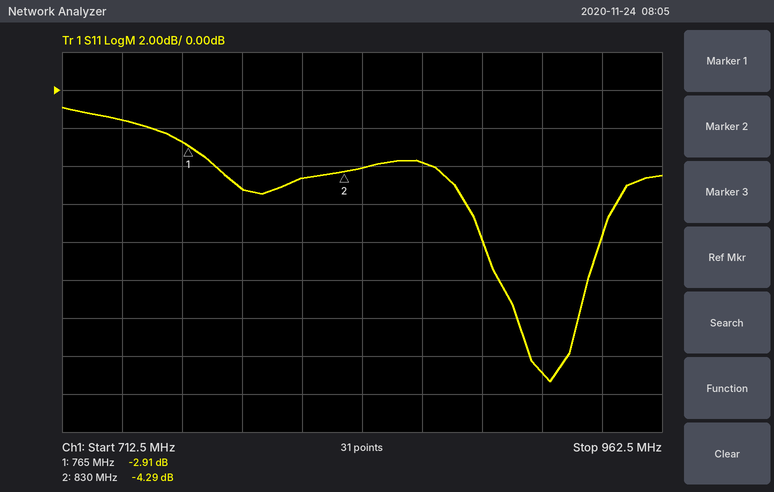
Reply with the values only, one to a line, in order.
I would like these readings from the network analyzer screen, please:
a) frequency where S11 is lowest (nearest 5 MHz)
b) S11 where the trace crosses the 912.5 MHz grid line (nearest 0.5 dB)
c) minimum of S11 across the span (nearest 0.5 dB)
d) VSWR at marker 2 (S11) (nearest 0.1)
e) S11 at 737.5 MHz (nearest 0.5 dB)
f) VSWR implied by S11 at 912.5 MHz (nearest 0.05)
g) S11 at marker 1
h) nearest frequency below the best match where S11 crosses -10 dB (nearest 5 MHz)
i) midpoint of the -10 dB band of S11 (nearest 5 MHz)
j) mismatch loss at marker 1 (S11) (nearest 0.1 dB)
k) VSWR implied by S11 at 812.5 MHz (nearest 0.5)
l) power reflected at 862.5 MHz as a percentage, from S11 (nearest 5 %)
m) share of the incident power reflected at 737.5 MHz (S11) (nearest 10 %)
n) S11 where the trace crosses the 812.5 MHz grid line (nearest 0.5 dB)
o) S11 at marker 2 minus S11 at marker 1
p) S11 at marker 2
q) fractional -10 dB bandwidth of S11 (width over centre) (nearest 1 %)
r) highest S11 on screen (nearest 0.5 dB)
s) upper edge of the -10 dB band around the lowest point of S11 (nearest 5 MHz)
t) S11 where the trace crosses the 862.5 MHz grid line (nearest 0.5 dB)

915 MHz
-15.0 dB
-15.5 dB
4.1
-1.5 dB
1.45
-2.91 dB
895 MHz
915 MHz
3.1 dB
4.0
40 %
70 %
-4.5 dB
-1.38 dB
-4.29 dB
4 %
-1.0 dB
930 MHz
-4.0 dB
